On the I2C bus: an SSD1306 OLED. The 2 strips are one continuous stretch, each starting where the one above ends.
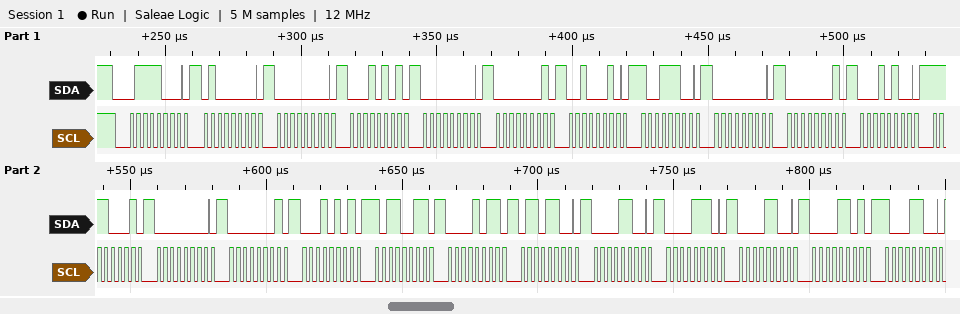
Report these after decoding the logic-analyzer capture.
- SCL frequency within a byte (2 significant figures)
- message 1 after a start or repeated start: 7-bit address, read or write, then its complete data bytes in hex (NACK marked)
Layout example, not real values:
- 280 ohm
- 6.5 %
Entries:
- 400 kHz
- 0x3C write: 40 00 15 00 01 22 9C 00 01 14 F1 00 01 15 B3 0B 6C 0C 0E 0C 0D 8C
